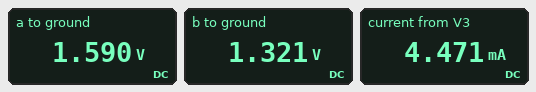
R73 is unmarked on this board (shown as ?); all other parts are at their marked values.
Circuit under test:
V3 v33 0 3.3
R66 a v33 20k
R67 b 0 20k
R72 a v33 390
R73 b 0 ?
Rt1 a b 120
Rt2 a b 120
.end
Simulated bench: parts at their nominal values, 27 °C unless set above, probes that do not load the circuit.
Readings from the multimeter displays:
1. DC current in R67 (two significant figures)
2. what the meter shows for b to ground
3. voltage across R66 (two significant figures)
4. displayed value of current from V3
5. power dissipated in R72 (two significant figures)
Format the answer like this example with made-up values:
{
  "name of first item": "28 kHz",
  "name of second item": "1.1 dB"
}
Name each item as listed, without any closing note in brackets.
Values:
{
  "DC current in R67": "66 µA",
  "what the meter shows for b to ground": "1.321 V",
  "voltage across R66": "1.7 V",
  "displayed value of current from V3": "4.471 mA",
  "power dissipated in R72": "7.5 mW"
}
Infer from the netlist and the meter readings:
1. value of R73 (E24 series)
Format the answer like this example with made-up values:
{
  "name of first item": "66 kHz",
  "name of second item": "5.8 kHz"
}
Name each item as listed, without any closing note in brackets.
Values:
{
  "value of R73": "300 Ω"
}
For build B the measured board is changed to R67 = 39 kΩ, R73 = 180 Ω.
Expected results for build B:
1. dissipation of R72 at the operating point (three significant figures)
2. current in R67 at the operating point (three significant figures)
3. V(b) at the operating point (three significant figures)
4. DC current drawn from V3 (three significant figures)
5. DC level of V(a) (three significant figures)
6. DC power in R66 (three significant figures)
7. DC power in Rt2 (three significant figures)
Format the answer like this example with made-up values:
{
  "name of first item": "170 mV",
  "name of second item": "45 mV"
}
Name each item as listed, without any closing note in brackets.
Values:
{
  "dissipation of R72 at the operating point": "10.6 mW",
  "current in R67 at the operating point": "24.4 µA",
  "V(b) at the operating point": "951 mV",
  "DC current drawn from V3": "5.31 mA",
  "DC level of V(a)": "1.27 V",
  "DC power in R66": "206 µW",
  "DC power in Rt2": "845 µW"
}
